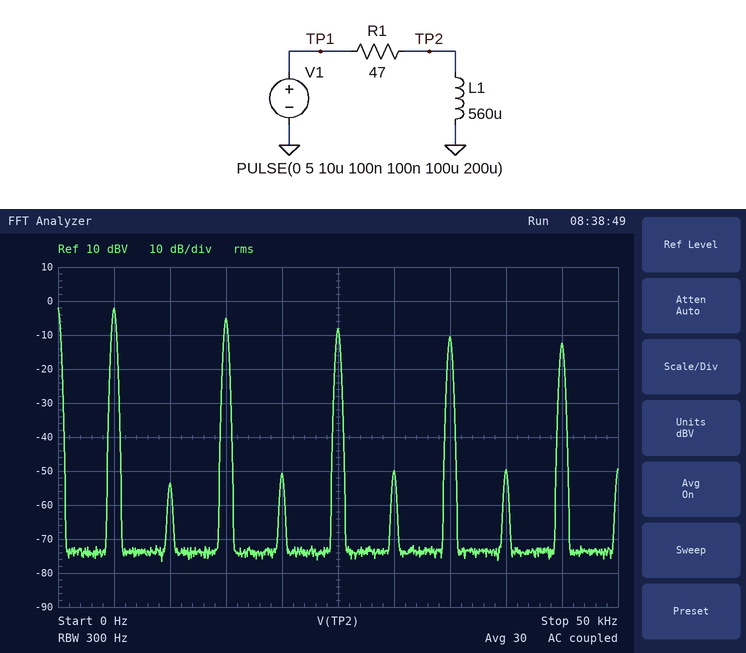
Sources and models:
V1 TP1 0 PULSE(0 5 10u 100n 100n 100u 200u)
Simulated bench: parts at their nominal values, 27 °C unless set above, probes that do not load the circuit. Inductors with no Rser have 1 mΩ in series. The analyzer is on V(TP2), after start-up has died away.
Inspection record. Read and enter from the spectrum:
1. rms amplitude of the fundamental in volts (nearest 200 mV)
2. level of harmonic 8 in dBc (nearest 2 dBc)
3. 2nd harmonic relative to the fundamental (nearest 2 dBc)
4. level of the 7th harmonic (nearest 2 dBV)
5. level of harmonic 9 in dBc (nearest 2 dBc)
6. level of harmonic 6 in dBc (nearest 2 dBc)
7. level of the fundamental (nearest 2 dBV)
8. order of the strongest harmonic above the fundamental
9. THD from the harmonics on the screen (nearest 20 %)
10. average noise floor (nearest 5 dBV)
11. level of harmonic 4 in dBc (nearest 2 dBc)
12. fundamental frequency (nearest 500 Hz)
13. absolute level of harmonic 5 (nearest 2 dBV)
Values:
800 mV
-48 dBc
-52 dBc
-10 dBV
-10 dBc
-48 dBc
-2 dBV
3
100 %
-75 dBV
-48 dBc
5.0 kHz
-8 dBV
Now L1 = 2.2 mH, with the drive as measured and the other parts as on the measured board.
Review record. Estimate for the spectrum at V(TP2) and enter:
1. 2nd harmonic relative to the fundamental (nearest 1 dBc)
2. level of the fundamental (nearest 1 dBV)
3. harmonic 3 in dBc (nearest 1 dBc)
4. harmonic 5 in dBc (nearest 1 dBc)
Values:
-55 dBc
5 dBV
-8 dBc
-12 dBc
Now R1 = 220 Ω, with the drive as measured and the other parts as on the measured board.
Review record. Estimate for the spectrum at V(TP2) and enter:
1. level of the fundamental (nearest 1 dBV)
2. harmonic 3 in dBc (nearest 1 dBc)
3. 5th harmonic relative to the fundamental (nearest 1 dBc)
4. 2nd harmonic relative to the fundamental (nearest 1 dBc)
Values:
-15 dBV
0 dBc
-1 dBc
-50 dBc
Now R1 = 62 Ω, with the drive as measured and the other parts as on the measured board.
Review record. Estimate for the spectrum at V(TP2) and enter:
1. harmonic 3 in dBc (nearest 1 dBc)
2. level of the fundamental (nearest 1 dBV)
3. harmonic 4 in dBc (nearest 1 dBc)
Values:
-2 dBc
-4 dBV
-47 dBc
